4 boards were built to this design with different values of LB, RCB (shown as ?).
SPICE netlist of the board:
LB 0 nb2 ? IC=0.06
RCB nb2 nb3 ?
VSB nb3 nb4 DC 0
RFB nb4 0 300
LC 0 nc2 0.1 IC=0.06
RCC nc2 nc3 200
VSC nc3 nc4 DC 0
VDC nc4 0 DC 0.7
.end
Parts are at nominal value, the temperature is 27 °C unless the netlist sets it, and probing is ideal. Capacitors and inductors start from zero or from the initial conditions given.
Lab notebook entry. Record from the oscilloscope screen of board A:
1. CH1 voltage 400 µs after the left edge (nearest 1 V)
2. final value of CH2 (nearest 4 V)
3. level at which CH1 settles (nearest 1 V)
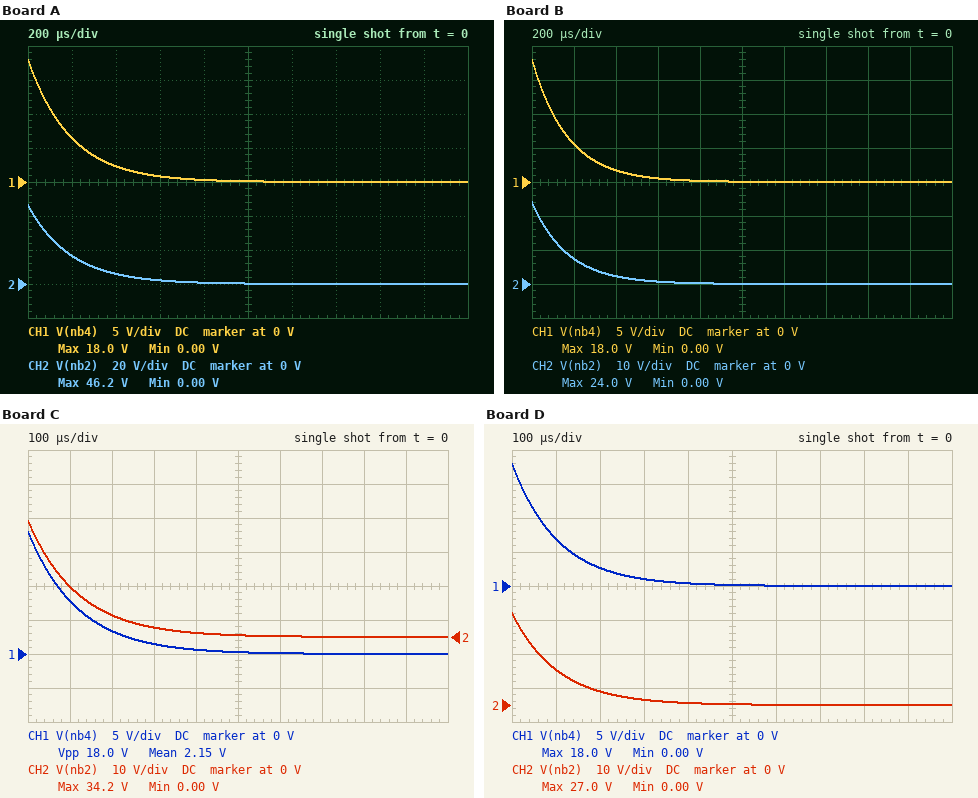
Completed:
2 V
0 V
0 V
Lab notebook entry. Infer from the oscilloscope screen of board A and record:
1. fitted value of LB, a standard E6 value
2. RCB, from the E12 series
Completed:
150 mH
470 Ω
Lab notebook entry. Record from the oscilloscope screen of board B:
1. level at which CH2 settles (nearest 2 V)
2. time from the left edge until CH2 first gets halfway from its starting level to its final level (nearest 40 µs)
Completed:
0 V
120 µs
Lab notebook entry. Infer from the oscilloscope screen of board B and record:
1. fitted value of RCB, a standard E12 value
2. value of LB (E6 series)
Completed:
100 Ω
68 mH
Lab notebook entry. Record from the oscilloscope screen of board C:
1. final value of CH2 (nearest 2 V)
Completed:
0 V
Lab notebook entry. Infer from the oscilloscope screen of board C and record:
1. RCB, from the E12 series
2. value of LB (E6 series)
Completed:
270 Ω
68 mH
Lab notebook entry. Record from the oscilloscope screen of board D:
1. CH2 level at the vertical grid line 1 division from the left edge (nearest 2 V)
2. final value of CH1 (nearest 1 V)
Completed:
10 V
0 V
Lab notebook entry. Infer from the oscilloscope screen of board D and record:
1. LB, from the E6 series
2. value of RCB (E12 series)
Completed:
47 mH
150 Ω
